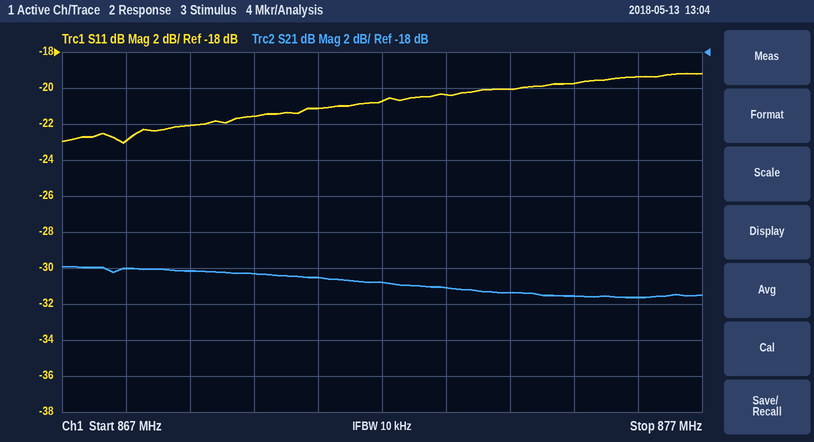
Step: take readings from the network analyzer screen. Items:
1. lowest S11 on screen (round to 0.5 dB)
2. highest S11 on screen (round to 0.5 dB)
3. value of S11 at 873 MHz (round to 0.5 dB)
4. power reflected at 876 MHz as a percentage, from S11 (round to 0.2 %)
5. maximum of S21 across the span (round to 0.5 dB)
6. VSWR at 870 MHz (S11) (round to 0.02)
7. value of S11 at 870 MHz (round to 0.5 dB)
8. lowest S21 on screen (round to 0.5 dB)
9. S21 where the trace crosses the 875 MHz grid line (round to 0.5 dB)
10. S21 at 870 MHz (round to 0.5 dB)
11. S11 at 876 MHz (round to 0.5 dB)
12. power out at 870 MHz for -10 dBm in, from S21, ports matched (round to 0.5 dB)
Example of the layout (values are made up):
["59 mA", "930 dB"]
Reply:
["-23.0 dB", "-19.0 dB", "-20.5 dB", "1.2 %", "-30.0 dB", "1.18", "-21.5 dB", "-31.5 dB", "-31.5 dB", "-30.5 dB", "-19.5 dB", "-40.5 dBm"]
